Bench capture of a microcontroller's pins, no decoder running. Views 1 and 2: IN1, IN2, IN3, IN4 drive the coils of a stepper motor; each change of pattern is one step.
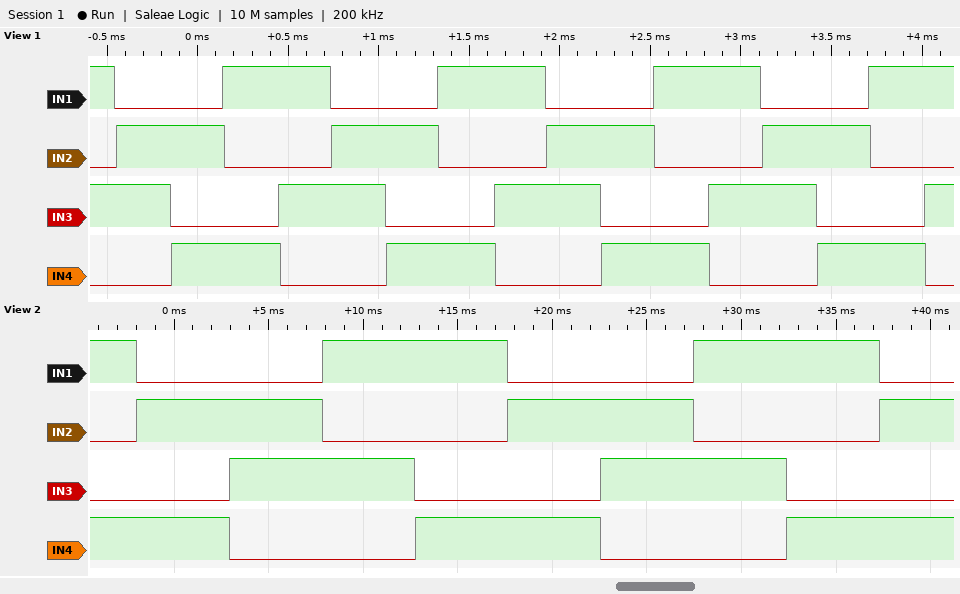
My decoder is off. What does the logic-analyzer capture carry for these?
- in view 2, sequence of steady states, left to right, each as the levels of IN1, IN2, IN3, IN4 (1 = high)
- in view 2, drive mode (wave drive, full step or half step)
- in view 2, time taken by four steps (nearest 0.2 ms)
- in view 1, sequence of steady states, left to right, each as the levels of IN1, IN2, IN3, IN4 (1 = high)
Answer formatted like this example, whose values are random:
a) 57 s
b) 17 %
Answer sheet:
a) 1001 0101 0110 1010 1001 0101 0110 1010 1001 0101
b) full step
c) 19.6 ms
d) 1010 0110 0101 1001 1010 0110 0101 1001 1010 0110 0101 1001 1010 0110 0101 1001 1010
